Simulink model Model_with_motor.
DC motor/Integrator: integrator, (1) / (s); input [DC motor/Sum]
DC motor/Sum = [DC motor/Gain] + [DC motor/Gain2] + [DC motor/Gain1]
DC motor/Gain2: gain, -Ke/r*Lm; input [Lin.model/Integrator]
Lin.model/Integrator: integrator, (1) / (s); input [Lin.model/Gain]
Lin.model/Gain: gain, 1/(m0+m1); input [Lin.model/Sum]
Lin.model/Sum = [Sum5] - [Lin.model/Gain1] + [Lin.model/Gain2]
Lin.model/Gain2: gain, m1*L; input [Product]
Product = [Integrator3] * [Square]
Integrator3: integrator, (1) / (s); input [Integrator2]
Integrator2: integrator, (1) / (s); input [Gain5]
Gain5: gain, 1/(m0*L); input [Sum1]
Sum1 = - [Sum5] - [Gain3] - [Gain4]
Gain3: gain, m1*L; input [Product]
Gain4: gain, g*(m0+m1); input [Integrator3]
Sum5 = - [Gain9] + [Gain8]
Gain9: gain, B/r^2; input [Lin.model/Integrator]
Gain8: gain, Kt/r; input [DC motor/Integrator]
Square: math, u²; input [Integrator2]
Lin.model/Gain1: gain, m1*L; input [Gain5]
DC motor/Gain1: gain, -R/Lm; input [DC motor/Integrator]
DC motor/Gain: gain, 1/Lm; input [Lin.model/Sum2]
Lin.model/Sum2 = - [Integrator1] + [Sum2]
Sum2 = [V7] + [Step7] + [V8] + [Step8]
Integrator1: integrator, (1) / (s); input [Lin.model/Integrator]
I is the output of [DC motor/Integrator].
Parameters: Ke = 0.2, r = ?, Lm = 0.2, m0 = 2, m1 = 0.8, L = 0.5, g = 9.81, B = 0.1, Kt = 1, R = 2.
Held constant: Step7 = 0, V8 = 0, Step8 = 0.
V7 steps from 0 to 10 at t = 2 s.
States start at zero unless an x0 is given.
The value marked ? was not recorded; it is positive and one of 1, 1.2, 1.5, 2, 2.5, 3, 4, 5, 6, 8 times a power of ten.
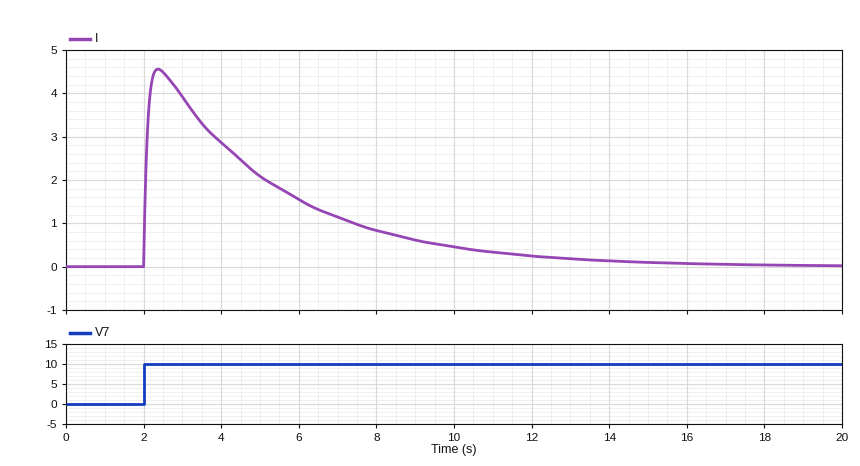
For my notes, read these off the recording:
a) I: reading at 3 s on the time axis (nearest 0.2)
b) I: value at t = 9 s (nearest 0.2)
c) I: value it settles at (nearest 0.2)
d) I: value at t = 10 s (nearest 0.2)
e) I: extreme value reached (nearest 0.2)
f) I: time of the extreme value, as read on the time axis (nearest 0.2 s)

4.0
0.6
0.0
0.4
4.6
2.4 s
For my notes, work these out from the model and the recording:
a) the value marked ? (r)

0.06
